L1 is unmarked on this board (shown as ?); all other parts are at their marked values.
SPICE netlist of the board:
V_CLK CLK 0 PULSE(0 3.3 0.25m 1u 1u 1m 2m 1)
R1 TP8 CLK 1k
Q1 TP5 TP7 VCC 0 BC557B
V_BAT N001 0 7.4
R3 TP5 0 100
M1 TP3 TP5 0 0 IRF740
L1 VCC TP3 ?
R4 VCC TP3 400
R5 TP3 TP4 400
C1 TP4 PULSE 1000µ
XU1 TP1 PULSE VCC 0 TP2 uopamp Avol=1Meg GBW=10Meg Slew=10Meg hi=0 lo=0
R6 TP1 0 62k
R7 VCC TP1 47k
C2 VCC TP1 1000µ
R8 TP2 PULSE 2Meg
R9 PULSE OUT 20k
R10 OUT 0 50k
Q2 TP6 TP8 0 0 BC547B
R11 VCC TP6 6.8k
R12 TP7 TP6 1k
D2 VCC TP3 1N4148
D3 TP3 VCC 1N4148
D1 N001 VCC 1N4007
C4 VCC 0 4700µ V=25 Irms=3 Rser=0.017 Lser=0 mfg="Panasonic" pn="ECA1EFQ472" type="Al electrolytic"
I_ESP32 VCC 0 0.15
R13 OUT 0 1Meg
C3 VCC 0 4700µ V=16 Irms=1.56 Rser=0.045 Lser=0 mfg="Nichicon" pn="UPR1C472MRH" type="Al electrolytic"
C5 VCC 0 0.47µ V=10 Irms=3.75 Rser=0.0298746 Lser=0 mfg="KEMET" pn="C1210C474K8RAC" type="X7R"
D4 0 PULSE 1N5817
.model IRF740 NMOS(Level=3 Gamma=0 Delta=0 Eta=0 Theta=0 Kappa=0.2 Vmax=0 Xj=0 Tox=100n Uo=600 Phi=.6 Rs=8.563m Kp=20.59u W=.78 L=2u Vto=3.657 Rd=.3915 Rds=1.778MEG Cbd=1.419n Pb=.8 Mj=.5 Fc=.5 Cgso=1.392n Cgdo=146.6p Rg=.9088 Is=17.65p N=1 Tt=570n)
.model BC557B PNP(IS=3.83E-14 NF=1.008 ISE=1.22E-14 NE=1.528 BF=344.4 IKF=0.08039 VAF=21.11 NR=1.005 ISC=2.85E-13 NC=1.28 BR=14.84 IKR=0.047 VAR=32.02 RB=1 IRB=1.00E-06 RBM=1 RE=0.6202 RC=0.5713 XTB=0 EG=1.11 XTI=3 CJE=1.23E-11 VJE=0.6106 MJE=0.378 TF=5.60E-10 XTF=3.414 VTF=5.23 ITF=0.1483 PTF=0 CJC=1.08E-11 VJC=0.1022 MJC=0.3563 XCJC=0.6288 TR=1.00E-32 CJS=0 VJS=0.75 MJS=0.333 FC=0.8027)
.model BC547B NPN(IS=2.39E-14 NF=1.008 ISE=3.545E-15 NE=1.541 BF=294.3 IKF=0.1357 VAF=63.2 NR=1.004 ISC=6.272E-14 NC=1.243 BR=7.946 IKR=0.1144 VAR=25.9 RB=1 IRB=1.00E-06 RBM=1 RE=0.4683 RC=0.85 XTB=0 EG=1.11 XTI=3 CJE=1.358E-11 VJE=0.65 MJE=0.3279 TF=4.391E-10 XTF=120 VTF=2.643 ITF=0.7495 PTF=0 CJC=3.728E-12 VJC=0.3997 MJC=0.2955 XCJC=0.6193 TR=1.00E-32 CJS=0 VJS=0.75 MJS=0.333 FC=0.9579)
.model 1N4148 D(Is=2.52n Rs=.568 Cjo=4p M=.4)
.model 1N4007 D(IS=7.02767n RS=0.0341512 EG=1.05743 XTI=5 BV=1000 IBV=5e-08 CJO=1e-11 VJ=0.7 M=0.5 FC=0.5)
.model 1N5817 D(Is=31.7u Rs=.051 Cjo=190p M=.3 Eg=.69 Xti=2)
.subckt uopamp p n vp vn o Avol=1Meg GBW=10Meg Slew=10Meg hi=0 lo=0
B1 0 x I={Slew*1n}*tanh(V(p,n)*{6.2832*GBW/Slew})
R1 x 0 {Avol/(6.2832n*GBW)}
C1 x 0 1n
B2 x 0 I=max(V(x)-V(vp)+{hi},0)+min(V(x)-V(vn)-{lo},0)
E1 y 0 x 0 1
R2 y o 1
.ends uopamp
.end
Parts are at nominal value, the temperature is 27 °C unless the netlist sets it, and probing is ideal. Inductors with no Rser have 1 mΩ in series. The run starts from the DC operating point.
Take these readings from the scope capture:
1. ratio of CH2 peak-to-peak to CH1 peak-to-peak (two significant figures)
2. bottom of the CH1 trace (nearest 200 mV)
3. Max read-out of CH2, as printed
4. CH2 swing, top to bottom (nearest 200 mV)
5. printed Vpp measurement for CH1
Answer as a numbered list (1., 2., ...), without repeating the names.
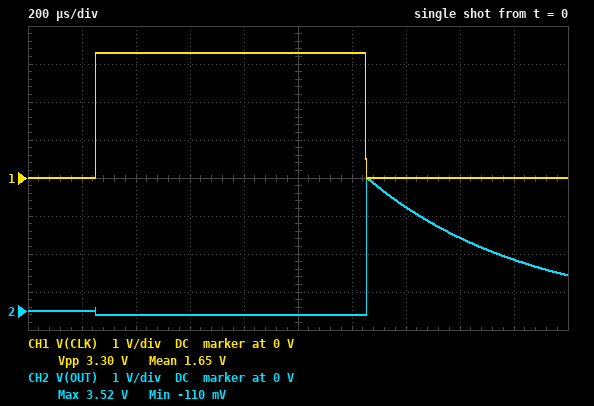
1. 1.1
2. 0 V
3. 3.52 V
4. 3.6 V
5. 3.30 V
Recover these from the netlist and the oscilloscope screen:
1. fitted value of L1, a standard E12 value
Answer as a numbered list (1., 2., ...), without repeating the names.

1. 330 µH
